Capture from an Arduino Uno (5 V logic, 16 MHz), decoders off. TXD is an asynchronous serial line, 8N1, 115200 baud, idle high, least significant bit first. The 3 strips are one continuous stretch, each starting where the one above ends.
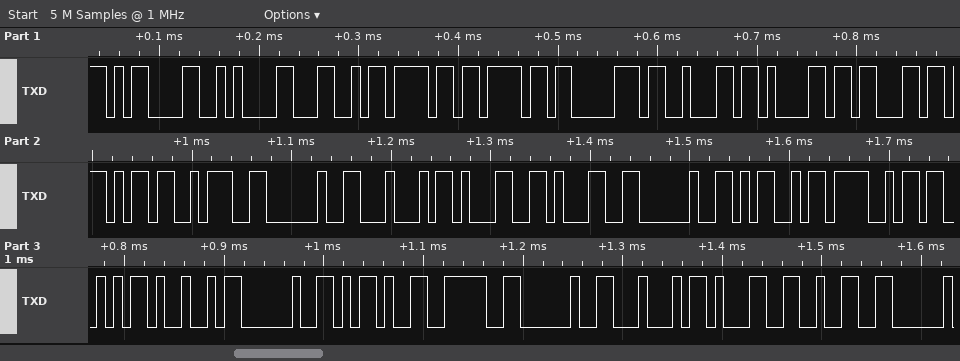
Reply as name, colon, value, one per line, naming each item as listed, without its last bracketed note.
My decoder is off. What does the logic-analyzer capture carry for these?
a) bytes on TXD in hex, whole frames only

bytes on TXD in hex, whole frames only: 0D 0A 4C 6F 6F 70 62 61 63 6B 3A 20 44 31 31 20 4D 4F 53 49 20 2D 3E 20 44 31 32
